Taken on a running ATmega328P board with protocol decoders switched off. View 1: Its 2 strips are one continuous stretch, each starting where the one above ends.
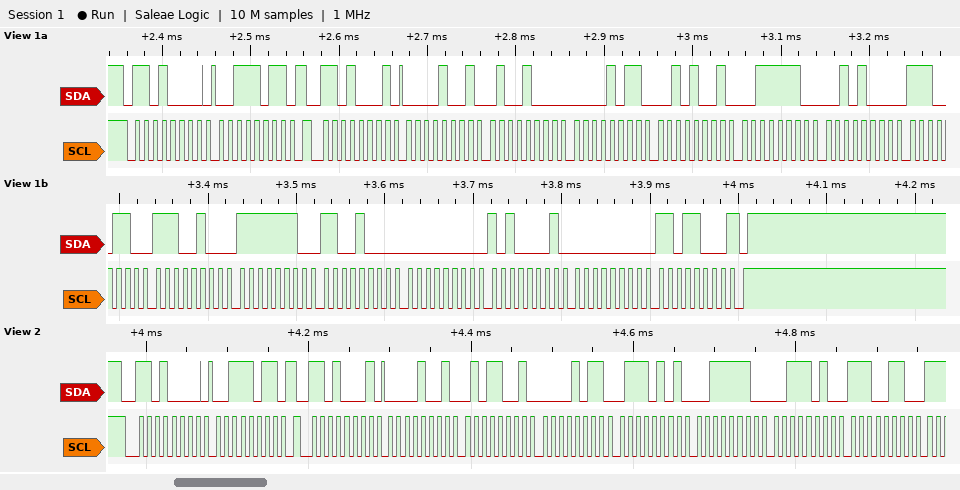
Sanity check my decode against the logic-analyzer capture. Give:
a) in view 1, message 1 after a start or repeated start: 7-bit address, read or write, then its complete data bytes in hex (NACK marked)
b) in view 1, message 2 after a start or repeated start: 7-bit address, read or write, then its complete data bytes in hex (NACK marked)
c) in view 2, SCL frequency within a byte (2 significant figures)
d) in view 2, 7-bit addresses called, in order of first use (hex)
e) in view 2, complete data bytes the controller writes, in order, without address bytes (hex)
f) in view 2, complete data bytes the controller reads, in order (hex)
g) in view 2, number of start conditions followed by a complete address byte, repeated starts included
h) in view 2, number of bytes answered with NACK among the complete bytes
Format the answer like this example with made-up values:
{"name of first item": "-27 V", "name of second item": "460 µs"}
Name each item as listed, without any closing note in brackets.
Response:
{"in view 1, message 1 after a start or repeated start: 7-bit address, read or write, then its complete data bytes in hex": "0x68 write: 3B", "in view 1, message 2 after a start or repeated start: 7-bit address, read or write, then its complete data bytes in hex": "0x68 read: 09 48 0B 29 3E 28 E6 E4 FE C8 00 A1 00 D8 NACK", "in view 2, SCL frequency within a byte": "100 kHz", "in view 2, 7-bit addresses called, in order of first use": "0x68", "in view 2, complete data bytes the controller writes, in order, without address bytes": "3B", "in view 2, complete data bytes the controller reads, in order": "09 59 0B 75 3E 3A E6", "in view 2, number of start conditions followed by a complete address byte, repeated starts included": "2", "in view 2, number of bytes answered with NACK among the complete bytes": "0"}
